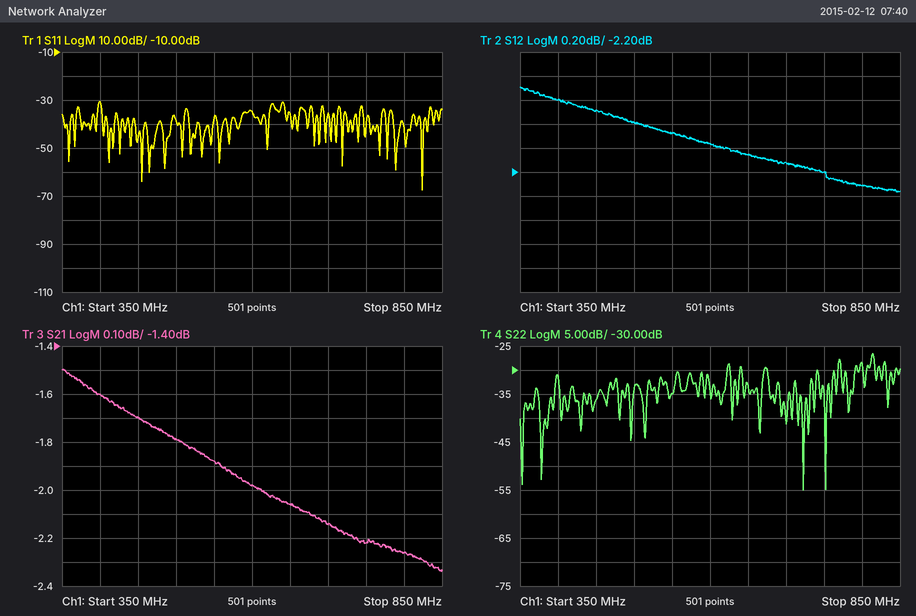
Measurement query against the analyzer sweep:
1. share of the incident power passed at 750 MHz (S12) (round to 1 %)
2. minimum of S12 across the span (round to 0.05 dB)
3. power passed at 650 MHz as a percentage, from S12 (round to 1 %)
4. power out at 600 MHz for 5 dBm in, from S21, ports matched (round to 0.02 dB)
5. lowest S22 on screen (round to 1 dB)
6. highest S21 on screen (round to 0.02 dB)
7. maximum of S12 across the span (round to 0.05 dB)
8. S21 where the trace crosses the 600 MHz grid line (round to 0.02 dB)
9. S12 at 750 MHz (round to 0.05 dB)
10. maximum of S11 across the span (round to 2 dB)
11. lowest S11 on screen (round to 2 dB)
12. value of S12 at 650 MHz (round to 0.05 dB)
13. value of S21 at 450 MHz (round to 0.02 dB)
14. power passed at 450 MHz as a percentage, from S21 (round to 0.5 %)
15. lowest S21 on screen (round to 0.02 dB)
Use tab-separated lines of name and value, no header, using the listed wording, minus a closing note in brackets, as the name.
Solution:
share of the incident power passed at 750 MHz (S12)	60 %
minimum of S12 across the span	-2.35 dB
power passed at 650 MHz as a percentage, from S12	62 %
power out at 600 MHz for 5 dBm in, from S21, ports matched	3.02 dBm
lowest S22 on screen	-55 dB
highest S21 on screen	-1.50 dB
maximum of S12 across the span	-1.50 dB
S21 where the trace crosses the 600 MHz grid line	-1.98 dB
S12 at 750 MHz	-2.20 dB
maximum of S11 across the span	-30 dB
lowest S11 on screen	-68 dB
value of S12 at 650 MHz	-2.05 dB
value of S21 at 450 MHz	-1.70 dB
power passed at 450 MHz as a percentage, from S21	67.5 %
lowest S21 on screen	-2.34 dB
